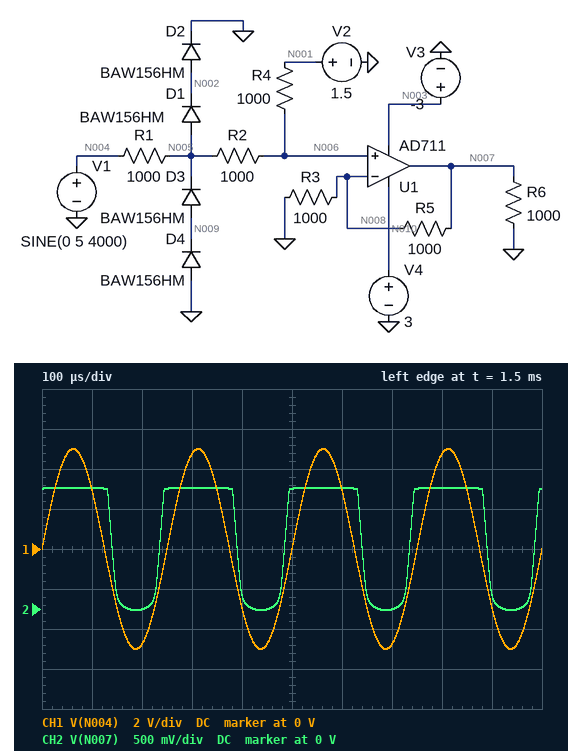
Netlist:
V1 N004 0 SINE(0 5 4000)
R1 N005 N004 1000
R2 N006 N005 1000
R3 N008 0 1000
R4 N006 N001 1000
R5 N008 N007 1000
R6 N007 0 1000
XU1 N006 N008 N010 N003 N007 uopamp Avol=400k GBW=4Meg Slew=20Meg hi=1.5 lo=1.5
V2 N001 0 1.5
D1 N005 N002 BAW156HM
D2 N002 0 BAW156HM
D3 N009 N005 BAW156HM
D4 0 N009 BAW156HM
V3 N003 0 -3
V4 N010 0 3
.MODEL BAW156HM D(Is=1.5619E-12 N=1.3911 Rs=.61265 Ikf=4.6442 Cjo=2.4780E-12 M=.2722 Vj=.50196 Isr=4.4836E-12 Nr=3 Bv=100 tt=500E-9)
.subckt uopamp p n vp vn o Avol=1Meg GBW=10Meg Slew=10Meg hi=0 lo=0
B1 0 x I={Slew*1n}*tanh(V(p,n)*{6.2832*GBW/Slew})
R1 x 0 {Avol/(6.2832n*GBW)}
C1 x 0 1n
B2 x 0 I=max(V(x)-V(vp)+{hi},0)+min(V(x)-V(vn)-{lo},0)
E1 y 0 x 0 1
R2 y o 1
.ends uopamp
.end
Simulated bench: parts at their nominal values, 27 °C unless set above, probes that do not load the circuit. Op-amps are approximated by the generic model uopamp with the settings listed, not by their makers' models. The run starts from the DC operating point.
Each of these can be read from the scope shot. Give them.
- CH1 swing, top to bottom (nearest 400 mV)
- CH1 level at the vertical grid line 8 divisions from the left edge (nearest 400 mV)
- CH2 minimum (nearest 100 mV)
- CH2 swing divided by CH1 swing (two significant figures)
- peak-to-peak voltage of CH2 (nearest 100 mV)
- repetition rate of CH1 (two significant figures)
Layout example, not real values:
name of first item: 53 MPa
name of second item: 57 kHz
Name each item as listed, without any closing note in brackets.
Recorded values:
CH1 swing, top to bottom: 10.0 V
CH1 level at the vertical grid line 8 divisions from the left edge: 4.8 V
CH2 minimum: 0 V
CH2 swing divided by CH1 swing: 0.15
peak-to-peak voltage of CH2: 1.5 V
repetition rate of CH1: 4.0 kHz
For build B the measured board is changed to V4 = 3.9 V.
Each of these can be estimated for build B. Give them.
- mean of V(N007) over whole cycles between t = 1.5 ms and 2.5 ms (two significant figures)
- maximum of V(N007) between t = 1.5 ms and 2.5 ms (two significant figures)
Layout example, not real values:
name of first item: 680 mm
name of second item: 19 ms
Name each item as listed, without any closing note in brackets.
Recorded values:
mean of V(N007) over whole cycles between t = 1.5 ms and 2.5 ms: 1.4 V
maximum of V(N007) between t = 1.5 ms and 2.5 ms: 2.4 V
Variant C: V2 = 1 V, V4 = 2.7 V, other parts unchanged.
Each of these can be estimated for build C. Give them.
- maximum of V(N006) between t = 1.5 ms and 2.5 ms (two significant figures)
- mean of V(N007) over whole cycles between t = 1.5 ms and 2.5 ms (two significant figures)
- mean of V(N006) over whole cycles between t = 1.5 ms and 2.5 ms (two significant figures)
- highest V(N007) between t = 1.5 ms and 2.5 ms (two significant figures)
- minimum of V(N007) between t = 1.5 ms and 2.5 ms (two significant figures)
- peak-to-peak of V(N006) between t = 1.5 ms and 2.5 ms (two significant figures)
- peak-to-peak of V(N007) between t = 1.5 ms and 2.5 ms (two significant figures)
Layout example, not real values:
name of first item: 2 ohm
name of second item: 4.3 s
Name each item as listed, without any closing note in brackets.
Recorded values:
maximum of V(N006) between t = 1.5 ms and 2.5 ms: 1.3 V
mean of V(N007) over whole cycles between t = 1.5 ms and 2.5 ms: 530 mV
mean of V(N006) over whole cycles between t = 1.5 ms and 2.5 ms: 550 mV
highest V(N007) between t = 1.5 ms and 2.5 ms: 1.2 V
minimum of V(N007) between t = 1.5 ms and 2.5 ms: -520 mV
peak-to-peak of V(N006) between t = 1.5 ms and 2.5 ms: 1.5 V
peak-to-peak of V(N007) between t = 1.5 ms and 2.5 ms: 1.7 V
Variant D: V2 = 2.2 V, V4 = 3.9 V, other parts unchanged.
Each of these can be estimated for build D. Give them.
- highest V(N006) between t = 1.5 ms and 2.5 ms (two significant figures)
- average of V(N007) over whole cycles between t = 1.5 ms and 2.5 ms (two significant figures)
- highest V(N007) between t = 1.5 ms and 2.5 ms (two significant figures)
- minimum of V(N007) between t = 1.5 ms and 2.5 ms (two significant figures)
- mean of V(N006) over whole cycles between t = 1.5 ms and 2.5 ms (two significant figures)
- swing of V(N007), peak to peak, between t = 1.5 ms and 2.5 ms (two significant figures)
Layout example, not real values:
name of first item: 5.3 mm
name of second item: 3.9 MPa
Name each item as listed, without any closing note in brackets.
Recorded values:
highest V(N006) between t = 1.5 ms and 2.5 ms: 1.9 V
average of V(N007) over whole cycles between t = 1.5 ms and 2.5 ms: 1.8 V
highest V(N007) between t = 1.5 ms and 2.5 ms: 2.4 V
minimum of V(N007) between t = 1.5 ms and 2.5 ms: 700 mV
mean of V(N006) over whole cycles between t = 1.5 ms and 2.5 ms: 1.2 V
swing of V(N007), peak to peak, between t = 1.5 ms and 2.5 ms: 1.7 V
